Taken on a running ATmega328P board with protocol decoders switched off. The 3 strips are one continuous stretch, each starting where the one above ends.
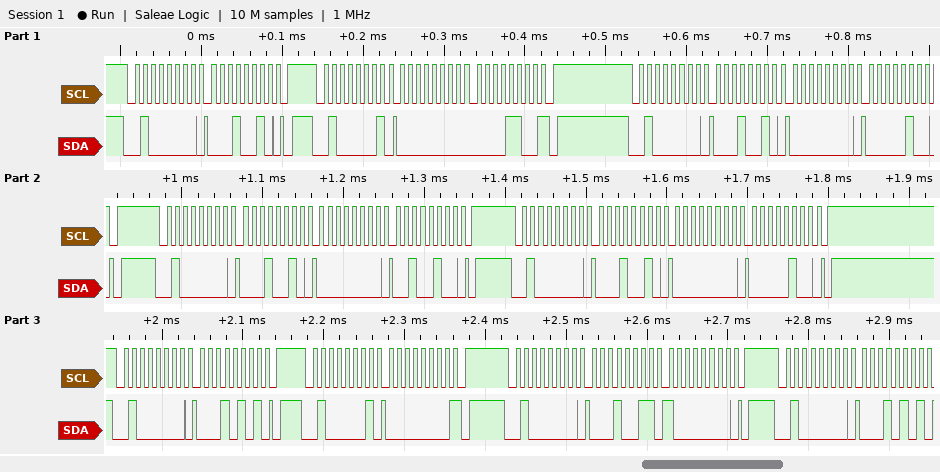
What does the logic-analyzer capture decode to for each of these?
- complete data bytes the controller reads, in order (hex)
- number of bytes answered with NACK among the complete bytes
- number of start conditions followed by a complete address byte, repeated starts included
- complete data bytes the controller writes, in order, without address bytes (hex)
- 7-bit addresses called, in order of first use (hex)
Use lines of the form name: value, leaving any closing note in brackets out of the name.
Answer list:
complete data bytes the controller reads, in order: 00 0C 00
number of bytes answered with NACK among the complete bytes: 2
number of start conditions followed by a complete address byte, repeated starts included: 9
complete data bytes the controller writes, in order, without address bytes: 12 12 00 04 12 00 24 12 00 04 15 13 80 15
7-bit addresses called, in order of first use: 0x20
